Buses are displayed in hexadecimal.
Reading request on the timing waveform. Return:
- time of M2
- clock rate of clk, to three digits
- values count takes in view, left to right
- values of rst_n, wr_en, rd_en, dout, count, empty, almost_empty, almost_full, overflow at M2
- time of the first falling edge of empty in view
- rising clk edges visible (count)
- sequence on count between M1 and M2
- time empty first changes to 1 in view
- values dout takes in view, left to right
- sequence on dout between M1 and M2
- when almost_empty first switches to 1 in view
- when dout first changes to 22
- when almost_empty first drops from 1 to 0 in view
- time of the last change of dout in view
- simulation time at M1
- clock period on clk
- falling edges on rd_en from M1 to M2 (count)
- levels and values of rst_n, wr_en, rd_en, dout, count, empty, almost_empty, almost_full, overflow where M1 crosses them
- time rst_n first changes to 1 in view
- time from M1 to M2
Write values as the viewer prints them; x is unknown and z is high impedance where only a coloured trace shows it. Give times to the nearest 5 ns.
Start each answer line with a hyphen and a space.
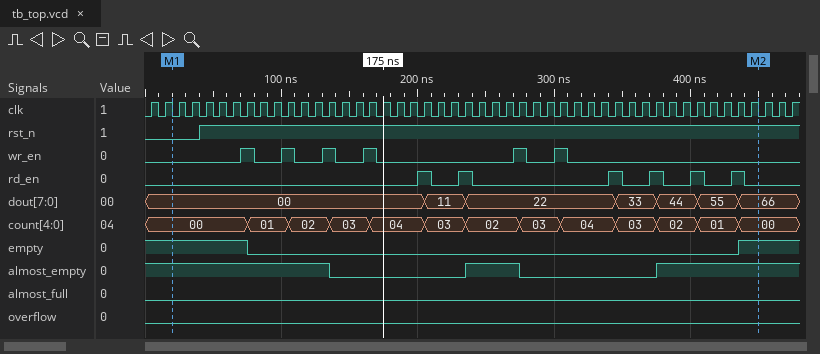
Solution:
- 450 ns
- 100 MHz
- 00, 01, 02, 03, 04, 03, 02, 03, 04, 03, 02, 01, 00
- rst_n=1, wr_en=0, rd_en=0, dout=66, count=00, empty=1, almost_empty=1, almost_full=0, overflow=0
- 75 ns
- 48
- 00, 01, 02, 03, 04, 03, 02, 03, 04, 03, 02, 01, 00
- 435 ns
- 00, 11, 22, 33, 44, 55, 66
- 00, 11, 22, 33, 44, 55, 66
- 235 ns
- 235 ns
- 135 ns
- 435 ns
- 20 ns
- 10 ns
- 6
- rst_n=0, wr_en=0, rd_en=0, dout=00, count=00, empty=1, almost_empty=1, almost_full=0, overflow=0
- 40 ns
- 430 ns
